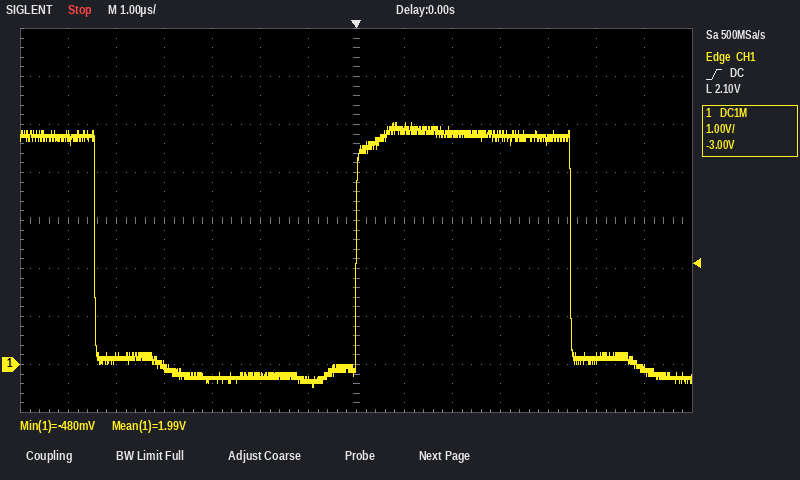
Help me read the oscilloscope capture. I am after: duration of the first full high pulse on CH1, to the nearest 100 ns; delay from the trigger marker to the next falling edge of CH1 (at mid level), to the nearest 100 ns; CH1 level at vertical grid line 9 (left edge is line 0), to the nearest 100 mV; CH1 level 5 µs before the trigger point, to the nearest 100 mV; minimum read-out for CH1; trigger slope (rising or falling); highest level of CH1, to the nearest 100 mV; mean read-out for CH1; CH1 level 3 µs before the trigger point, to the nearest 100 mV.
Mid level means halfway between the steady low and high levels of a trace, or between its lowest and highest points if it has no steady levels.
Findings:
4.5 µs
4.5 µs
4.8 V
200 mV
-480 mV
rising
5.0 V
1.99 V
-300 mV
